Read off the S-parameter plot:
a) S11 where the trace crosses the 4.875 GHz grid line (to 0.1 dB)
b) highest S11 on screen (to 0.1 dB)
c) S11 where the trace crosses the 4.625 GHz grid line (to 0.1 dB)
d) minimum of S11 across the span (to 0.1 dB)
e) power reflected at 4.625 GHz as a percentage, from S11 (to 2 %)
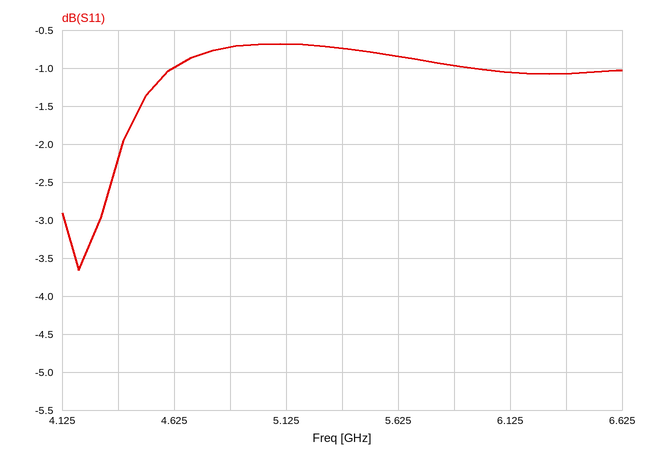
-0.7 dB
-0.7 dB
-1.0 dB
-3.7 dB
80 %
